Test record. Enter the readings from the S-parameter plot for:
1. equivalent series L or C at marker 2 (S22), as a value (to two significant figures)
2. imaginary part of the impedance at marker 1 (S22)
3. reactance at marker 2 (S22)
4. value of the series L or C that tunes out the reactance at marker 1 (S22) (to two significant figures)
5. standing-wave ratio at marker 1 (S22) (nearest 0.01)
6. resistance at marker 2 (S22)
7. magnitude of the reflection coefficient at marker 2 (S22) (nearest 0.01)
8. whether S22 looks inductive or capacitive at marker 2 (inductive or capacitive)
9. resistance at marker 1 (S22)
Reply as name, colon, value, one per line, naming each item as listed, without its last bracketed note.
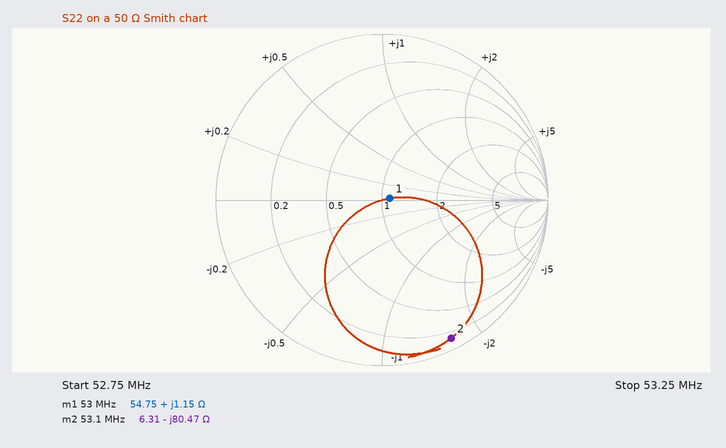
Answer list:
equivalent series L or C at marker 2 (S22), as a value: 37 pF
imaginary part of the impedance at marker 1: +1.15 Ω
reactance at marker 2: -80.47 Ω
value of the series L or C that tunes out the reactance at marker 1 (S22): 2.6 nF
standing-wave ratio at marker 1 (S22): 1.10
resistance at marker 2: 6.31 Ω
magnitude of the reflection coefficient at marker 2 (S22): 0.93
whether S22 looks inductive or capacitive at marker 2: capacitive
resistance at marker 1: 54.75 Ω
